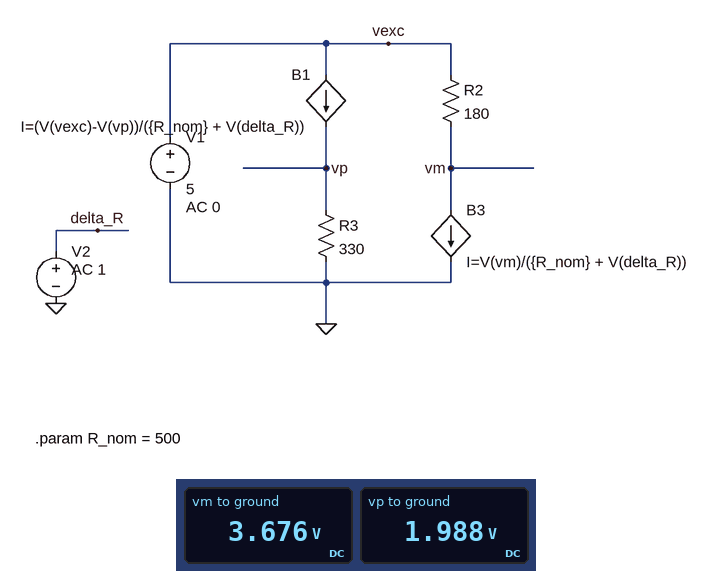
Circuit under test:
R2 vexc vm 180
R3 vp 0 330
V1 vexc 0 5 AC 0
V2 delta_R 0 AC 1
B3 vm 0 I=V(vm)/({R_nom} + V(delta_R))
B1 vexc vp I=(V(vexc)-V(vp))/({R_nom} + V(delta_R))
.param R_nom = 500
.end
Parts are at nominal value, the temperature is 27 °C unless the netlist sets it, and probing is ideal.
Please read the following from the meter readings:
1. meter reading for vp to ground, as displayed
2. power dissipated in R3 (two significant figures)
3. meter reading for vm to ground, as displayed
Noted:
1.988 V
12 mW
3.676 V
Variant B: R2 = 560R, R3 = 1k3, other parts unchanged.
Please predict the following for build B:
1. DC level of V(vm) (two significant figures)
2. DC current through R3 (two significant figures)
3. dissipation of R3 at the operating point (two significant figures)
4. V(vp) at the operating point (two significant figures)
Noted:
2.4 V
2.8 mA
10 mW
3.6 V
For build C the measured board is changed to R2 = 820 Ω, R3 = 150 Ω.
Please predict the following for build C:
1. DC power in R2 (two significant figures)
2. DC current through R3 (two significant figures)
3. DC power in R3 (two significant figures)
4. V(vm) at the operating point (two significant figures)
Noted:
12 mW
7.7 mA
8.9 mW
1.9 V
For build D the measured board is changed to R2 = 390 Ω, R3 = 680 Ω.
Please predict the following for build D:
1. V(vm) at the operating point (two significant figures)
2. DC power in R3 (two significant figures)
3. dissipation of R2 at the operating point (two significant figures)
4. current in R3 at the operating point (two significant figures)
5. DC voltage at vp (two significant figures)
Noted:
2.8 V
12 mW
12 mW
4.2 mA
2.9 V
